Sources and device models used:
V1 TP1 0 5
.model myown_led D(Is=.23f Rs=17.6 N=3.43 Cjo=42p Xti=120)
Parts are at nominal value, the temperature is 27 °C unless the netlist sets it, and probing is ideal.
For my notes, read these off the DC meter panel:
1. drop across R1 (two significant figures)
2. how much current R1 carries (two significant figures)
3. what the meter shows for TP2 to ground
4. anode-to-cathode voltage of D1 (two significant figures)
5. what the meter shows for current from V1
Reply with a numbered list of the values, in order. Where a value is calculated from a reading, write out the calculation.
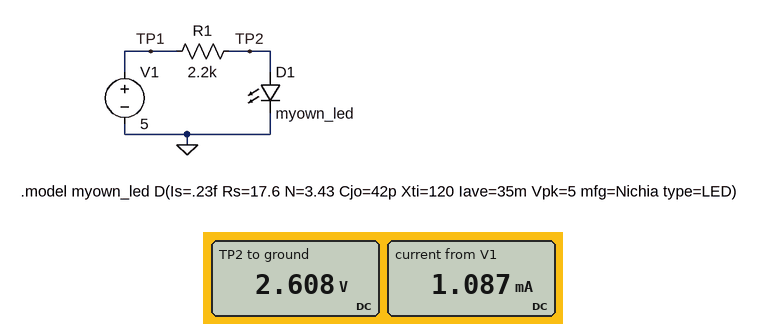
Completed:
1. 5 V - 2.608 V = 2.4 V
2. (5 V - 2.608 V) / 2.2 kΩ = 1.1 mA
3. 2.608 V
4. 2.608 V = 2.6 V
5. 1.087 mA
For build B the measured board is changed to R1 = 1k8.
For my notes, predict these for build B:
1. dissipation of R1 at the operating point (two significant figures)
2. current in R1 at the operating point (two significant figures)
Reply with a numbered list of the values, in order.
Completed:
1. 3.1 mW
2. 1.3 mA
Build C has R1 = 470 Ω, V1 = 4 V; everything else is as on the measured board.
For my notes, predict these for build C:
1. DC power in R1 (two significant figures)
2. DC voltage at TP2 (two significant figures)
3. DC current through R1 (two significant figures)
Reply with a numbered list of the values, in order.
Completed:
1. 3.5 mW
2. 2.7 V
3. 2.7 mA
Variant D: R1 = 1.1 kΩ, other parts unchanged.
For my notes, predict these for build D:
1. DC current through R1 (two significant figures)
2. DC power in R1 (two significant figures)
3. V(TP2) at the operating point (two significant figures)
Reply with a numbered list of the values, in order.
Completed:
1. 2.1 mA
2. 4.9 mW
3. 2.7 V
